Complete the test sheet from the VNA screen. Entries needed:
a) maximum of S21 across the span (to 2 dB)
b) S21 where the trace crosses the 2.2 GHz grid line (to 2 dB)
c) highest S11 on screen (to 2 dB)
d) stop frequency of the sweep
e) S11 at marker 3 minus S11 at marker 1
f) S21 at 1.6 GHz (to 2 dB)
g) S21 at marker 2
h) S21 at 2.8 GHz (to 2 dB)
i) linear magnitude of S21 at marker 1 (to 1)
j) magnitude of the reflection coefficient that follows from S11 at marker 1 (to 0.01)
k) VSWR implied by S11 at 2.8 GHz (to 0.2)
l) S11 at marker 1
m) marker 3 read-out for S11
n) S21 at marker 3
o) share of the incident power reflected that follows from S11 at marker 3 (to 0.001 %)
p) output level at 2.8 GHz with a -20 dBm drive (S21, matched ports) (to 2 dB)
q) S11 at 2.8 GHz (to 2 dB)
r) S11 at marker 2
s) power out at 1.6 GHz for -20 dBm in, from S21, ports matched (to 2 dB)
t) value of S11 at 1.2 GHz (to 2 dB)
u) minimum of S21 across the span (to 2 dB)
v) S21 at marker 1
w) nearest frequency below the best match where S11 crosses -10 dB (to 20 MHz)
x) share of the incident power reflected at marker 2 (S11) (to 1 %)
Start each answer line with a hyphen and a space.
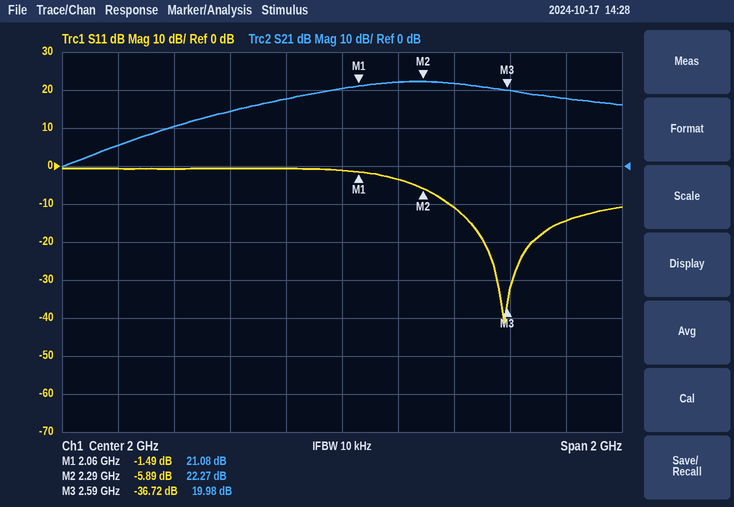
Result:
- 22 dB
- 22 dB
- 0 dB
- 3 GHz
- -35.23 dB
- 14 dB
- 22.27 dB
- 18 dB
- 11
- 0.84
- 1.4
- -1.49 dB
- -36.72 dB
- 19.98 dB
- 0.021 %
- -2 dBm
- -14 dB
- -5.89 dB
- -6 dBm
- 0 dB
- 0 dB
- 21.08 dB
- 2.38 GHz
- 26 %
